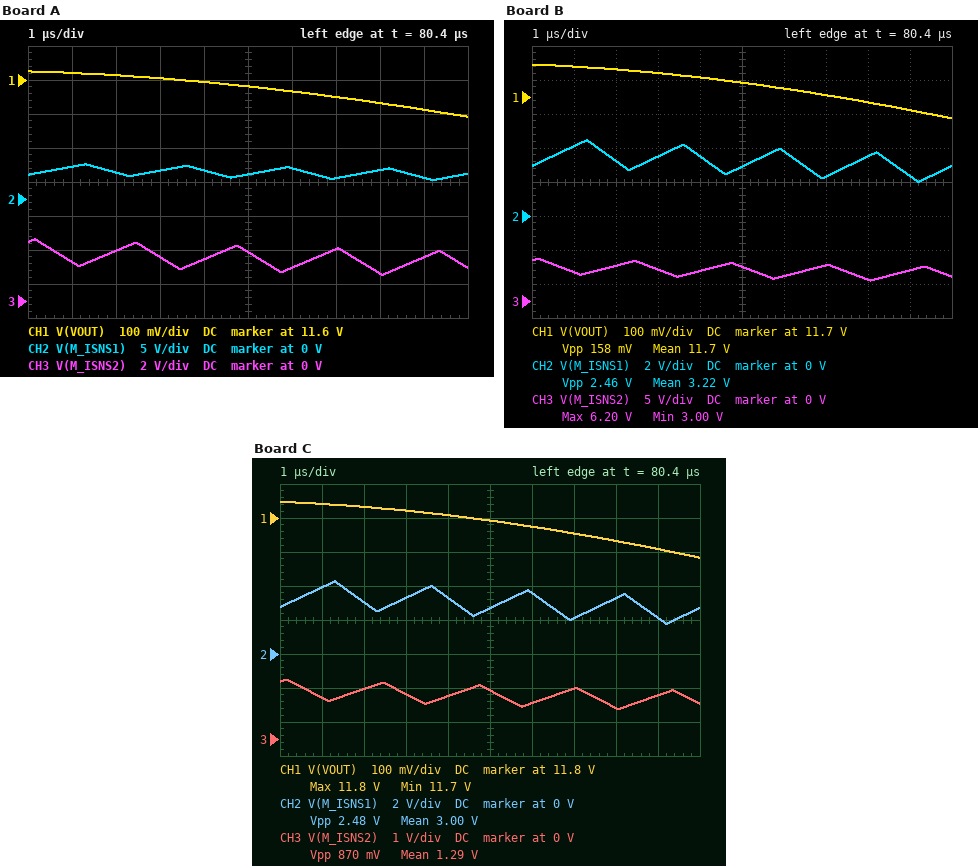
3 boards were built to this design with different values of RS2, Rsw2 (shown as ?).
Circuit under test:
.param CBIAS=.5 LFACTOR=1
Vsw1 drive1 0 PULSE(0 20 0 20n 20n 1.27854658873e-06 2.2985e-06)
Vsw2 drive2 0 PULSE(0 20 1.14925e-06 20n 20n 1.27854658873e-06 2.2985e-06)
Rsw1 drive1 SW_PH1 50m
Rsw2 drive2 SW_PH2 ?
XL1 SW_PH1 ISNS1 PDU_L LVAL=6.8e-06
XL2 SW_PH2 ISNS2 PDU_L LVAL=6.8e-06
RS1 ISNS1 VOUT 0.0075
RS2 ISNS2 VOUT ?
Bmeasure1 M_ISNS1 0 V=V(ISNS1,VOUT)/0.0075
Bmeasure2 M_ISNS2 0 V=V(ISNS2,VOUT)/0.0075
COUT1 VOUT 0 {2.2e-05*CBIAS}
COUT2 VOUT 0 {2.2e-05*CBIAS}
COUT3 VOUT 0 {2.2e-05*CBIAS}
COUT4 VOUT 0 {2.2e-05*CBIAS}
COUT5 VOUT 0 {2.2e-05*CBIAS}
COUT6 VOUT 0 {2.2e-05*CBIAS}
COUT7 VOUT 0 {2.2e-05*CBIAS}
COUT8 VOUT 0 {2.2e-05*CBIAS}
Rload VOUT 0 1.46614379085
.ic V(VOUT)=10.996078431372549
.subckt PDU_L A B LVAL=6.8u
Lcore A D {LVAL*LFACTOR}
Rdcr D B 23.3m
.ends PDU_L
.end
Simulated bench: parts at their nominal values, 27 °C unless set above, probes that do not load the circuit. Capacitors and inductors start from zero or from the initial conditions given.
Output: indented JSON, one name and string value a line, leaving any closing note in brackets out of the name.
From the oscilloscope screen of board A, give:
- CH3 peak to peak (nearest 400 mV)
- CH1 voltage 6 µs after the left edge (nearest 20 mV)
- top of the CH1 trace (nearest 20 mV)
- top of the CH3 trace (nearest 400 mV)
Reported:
{
  "CH3 peak to peak": "2.0 V",
  "CH1 voltage 6 µs after the left edge": "11.56 V",
  "top of the CH1 trace": "11.62 V",
  "top of the CH3 trace": "3.6 V"
}
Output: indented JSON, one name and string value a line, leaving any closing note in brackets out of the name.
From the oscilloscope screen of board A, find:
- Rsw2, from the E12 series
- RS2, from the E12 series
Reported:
{
  "Rsw2, from the E12 series": "0.068 Ω",
  "RS2, from the E12 series": "6.8 mΩ"
}
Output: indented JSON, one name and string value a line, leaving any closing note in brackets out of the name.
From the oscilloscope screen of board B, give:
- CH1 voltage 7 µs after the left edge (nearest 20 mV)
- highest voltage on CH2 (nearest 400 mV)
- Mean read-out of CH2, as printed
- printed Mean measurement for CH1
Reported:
{
  "CH1 voltage 7 µs after the left edge": "11.70 V",
  "highest voltage on CH2": "4.4 V",
  "Mean read-out of CH2, as printed": "3.22 V",
  "printed Mean measurement for CH1": "11.7 V"
}
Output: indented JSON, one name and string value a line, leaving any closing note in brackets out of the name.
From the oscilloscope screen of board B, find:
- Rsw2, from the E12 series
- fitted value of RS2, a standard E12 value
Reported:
{
  "Rsw2, from the E12 series": "0.022 Ω",
  "fitted value of RS2, a standard E12 value": "0.01 Ω"
}
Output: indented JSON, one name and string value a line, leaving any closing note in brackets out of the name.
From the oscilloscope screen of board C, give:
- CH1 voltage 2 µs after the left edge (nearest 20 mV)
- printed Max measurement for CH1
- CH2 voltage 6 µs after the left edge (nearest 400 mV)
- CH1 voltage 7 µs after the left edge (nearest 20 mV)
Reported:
{
  "CH1 voltage 2 µs after the left edge": "11.84 V",
  "printed Max measurement for CH1": "11.8 V",
  "CH2 voltage 6 µs after the left edge": "3.6 V",
  "CH1 voltage 7 µs after the left edge": "11.76 V"
}
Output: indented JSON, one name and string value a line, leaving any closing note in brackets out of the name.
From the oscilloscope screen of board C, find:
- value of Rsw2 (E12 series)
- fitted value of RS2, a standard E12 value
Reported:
{
  "value of Rsw2": "0.018 Ω",
  "fitted value of RS2, a standard E12 value": "2.7 mΩ"
}
